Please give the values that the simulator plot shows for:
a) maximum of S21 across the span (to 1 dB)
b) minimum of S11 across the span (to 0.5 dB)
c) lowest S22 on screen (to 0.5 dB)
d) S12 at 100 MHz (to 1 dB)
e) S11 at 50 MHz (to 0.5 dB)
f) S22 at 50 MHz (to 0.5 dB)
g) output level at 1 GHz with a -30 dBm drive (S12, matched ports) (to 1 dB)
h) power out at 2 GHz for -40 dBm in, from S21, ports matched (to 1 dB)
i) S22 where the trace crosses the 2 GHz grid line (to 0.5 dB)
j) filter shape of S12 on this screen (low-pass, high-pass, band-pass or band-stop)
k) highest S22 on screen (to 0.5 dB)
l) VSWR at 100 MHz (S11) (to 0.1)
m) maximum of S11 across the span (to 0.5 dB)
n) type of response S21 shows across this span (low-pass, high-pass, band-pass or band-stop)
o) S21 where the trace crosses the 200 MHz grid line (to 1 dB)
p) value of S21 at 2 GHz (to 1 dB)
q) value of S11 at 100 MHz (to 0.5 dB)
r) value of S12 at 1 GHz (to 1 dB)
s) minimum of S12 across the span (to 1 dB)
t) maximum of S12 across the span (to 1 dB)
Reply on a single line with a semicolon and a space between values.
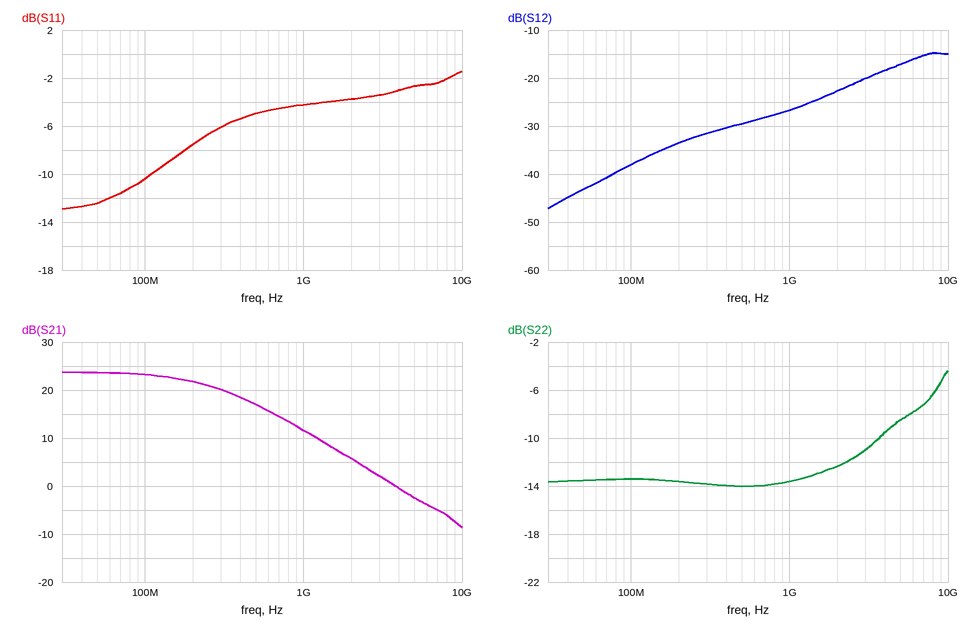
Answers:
24 dB; -13.0 dB; -14.0 dB; -38 dB; -12.5 dB; -13.5 dB; -57 dBm; -34 dBm; -12.5 dB; high-pass; -4.5 dB; 1.9; -1.5 dB; low-pass; 22 dB; 6 dB; -10.5 dB; -27 dB; -47 dB; -15 dB
